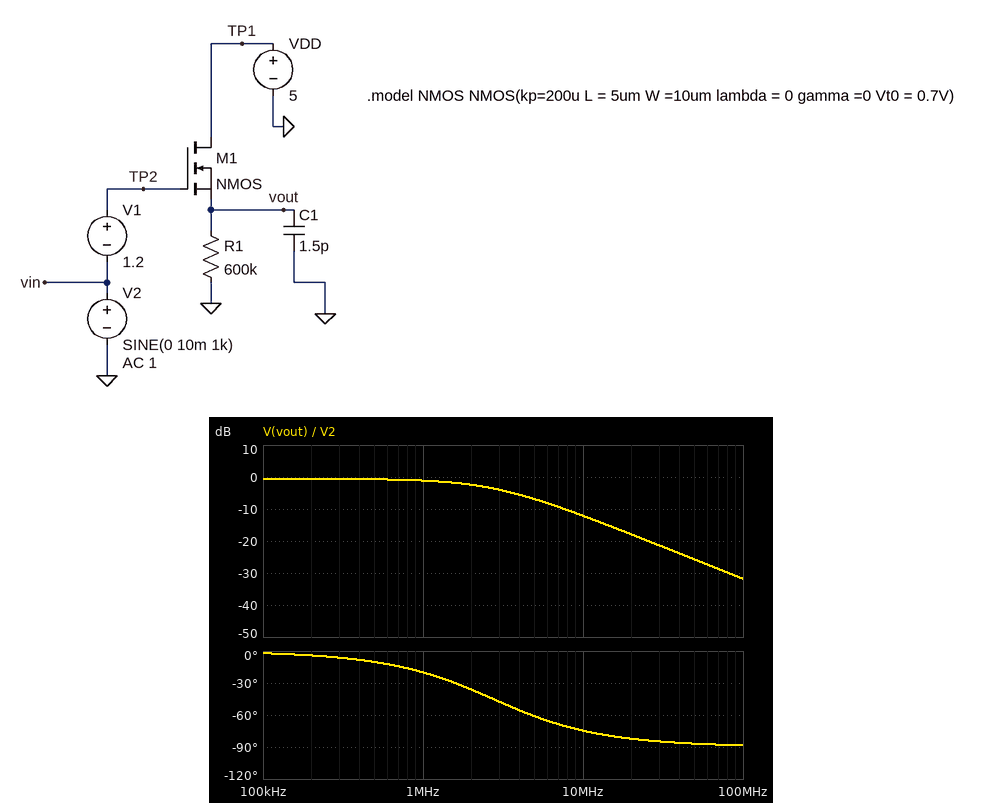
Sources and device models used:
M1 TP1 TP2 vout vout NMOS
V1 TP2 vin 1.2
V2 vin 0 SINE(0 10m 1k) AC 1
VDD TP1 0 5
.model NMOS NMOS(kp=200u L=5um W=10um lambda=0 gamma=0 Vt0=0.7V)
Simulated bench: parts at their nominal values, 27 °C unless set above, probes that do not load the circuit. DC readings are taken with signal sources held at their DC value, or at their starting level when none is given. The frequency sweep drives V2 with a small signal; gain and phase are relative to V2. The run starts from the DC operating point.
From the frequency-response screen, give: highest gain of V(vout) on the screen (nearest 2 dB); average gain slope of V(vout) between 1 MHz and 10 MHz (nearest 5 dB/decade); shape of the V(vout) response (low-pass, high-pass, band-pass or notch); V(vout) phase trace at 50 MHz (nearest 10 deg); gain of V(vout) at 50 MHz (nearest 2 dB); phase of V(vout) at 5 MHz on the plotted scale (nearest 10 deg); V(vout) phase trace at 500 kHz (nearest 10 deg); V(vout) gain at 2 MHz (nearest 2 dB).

0 dB
-10 dB/decade
low-pass
-90 deg
-26 dB
-60 deg
-10 deg
-2 dB
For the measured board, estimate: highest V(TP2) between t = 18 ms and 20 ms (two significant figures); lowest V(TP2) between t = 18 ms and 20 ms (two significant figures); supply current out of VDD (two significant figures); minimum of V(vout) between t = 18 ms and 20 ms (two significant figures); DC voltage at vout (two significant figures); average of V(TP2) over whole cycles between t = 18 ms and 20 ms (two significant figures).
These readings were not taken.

1.2 V
1.2 V
730 nA
430 mV
440 mV
1.2 V
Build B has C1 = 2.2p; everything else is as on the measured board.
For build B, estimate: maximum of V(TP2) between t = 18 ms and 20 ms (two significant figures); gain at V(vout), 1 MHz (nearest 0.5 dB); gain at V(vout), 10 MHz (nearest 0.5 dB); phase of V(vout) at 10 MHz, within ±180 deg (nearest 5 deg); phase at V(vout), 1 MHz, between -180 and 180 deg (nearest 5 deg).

1.2 V
-1.5 dB
-15.5 dB
-80 deg
-30 deg
